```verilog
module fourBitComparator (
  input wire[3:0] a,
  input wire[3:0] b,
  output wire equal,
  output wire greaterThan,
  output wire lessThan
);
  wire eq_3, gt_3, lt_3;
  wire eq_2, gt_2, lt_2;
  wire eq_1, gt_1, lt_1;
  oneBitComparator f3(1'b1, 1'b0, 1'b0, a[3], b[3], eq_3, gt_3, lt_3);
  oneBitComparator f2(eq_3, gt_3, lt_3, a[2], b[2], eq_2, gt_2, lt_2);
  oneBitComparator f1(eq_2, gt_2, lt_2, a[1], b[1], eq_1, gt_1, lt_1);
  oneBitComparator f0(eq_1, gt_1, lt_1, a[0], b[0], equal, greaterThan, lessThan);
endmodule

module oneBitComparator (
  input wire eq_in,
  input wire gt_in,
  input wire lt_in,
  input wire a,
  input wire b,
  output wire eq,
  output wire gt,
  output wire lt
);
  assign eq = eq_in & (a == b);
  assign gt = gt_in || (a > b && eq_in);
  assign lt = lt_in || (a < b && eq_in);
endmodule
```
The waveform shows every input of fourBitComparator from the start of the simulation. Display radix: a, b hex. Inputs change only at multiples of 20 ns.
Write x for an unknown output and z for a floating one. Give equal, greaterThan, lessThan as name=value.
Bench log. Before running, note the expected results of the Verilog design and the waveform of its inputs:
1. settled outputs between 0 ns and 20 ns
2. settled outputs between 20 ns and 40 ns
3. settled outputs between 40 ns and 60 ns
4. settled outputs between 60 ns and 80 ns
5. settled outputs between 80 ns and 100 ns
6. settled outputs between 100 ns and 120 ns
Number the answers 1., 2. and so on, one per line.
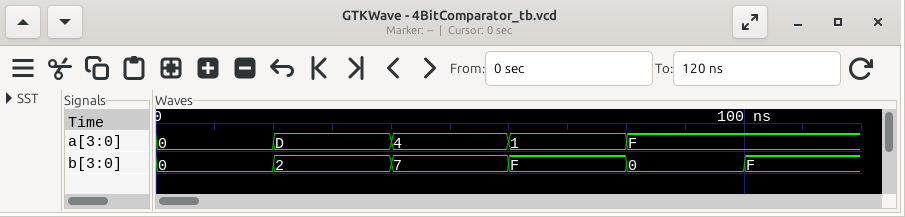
1. equal=1, greaterThan=0, lessThan=0
2. equal=0, greaterThan=1, lessThan=0
3. equal=0, greaterThan=0, lessThan=1
4. equal=0, greaterThan=0, lessThan=1
5. equal=0, greaterThan=1, lessThan=0
6. equal=1, greaterThan=0, lessThan=0
